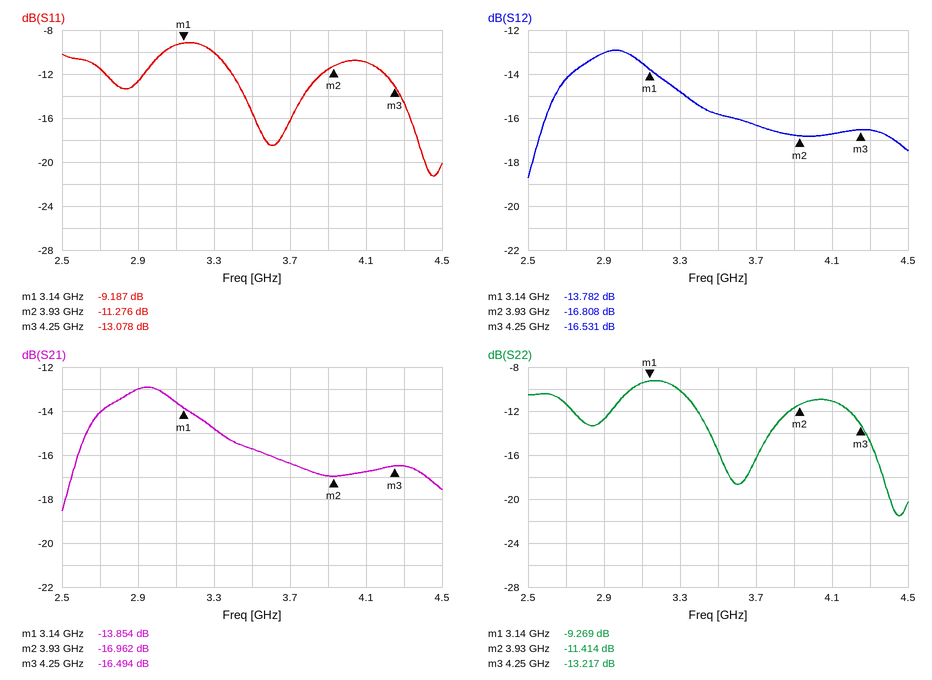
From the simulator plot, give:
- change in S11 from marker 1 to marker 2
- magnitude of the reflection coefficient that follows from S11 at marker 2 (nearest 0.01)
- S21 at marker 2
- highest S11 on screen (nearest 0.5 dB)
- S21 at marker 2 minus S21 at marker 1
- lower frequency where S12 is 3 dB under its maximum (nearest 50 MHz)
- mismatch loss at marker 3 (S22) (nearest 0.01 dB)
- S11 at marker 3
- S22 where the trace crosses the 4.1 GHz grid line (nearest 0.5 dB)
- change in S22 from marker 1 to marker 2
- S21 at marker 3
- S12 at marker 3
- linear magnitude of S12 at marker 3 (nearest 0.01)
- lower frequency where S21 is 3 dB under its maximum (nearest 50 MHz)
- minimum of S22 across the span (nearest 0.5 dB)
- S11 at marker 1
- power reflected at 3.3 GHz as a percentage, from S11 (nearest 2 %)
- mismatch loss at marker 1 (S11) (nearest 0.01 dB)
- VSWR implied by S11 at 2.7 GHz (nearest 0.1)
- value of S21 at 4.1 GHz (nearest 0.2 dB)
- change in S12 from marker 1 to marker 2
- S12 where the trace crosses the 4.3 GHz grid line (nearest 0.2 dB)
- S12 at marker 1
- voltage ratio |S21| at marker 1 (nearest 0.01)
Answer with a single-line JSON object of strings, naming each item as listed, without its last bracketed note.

{"change in S11 from marker 1 to marker 2": "-2.089 dB", "magnitude of the reflection coefficient that follows from S11 at marker 2": "0.27", "S21 at marker 2": "-16.962 dB", "highest S11 on screen": "-9.0 dB", "S21 at marker 2 minus S21 at marker 1": "-3.108 dB", "lower frequency where S12 is 3 dB under its maximum": "2.60 GHz", "mismatch loss at marker 3 (S22)": "0.21 dB", "S11 at marker 3": "-13.078 dB", "S22 where the trace crosses the 4.1 GHz grid line": "-11.0 dB", "change in S22 from marker 1 to marker 2": "-2.145 dB", "S21 at marker 3": "-16.494 dB", "S12 at marker 3": "-16.531 dB", "linear magnitude of S12 at marker 3": "0.15", "lower frequency where S21 is 3 dB under its maximum": "2.60 GHz", "minimum of S22 across the span": "-21.5 dB", "S11 at marker 1": "-9.187 dB", "power reflected at 3.3 GHz as a percentage, from S11": "10 %", "mismatch loss at marker 1 (S11)": "0.56 dB", "VSWR implied by S11 at 2.7 GHz": "1.7", "value of S21 at 4.1 GHz": "-16.8 dB", "change in S12 from marker 1 to marker 2": "-3.026 dB", "S12 where the trace crosses the 4.3 GHz grid line": "-16.6 dB", "S12 at marker 1": "-13.782 dB", "voltage ratio |S21| at marker 1": "0.20"}
